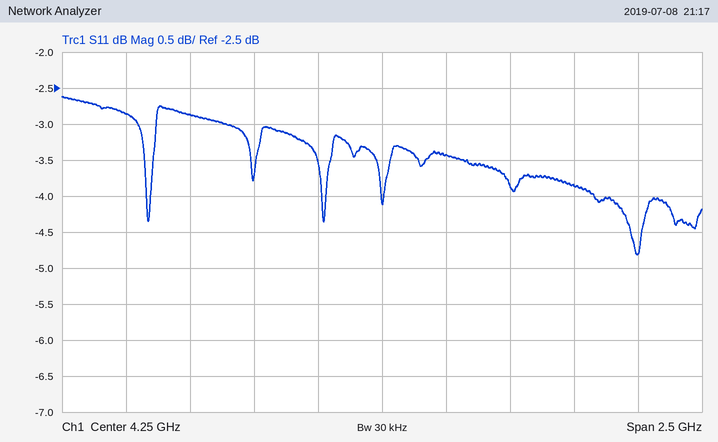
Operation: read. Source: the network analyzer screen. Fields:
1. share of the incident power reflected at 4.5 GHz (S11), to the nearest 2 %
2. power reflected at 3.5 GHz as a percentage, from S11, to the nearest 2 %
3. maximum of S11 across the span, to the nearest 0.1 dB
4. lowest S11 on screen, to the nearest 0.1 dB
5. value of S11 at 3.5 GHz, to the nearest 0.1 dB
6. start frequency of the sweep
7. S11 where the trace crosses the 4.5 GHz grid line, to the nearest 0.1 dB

46 %
52 %
-2.6 dB
-4.8 dB
-2.9 dB
3 GHz
-3.4 dB
